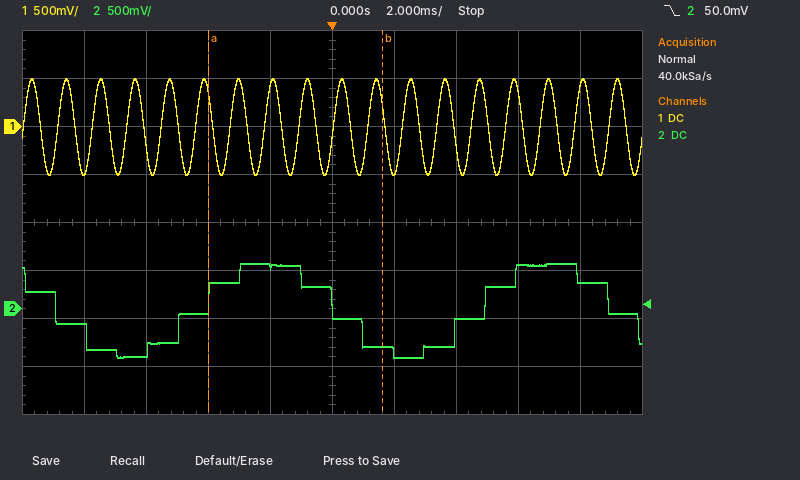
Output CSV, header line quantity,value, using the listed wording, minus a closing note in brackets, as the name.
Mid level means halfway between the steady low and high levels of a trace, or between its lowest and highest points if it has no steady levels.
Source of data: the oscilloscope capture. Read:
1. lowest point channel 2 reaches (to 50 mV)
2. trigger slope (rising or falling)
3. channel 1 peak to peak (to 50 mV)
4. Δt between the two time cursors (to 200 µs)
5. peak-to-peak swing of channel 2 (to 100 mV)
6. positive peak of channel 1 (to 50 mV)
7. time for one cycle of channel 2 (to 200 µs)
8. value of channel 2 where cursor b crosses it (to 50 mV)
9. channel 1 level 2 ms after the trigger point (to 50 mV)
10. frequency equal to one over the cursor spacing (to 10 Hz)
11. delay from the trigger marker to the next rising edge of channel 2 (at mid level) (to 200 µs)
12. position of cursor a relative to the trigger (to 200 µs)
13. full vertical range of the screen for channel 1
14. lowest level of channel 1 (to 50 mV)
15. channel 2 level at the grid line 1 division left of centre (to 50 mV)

quantity,value
lowest point channel 2 reaches,-500 mV
trigger slope,falling
channel 1 peak to peak,1.00 V
Δt between the two time cursors,5.6 ms
peak-to-peak swing of channel 2,1.00 V
positive peak of channel 1,500 mV
time for one cycle of channel 2,9.0 ms
value of channel 2 where cursor b crosses it,-400 mV
channel 1 level 2 ms after the trigger point,-450 mV
frequency equal to one over the cursor spacing,180 Hz
delay from the trigger marker to the next rising edge of channel 2 (at mid level),5.0 ms
position of cursor a relative to the trigger,-4.0 ms
full vertical range of the screen for channel 1,4 V
lowest level of channel 1,-500 mV
channel 2 level at the grid line 1 division left of centre,450 mV
